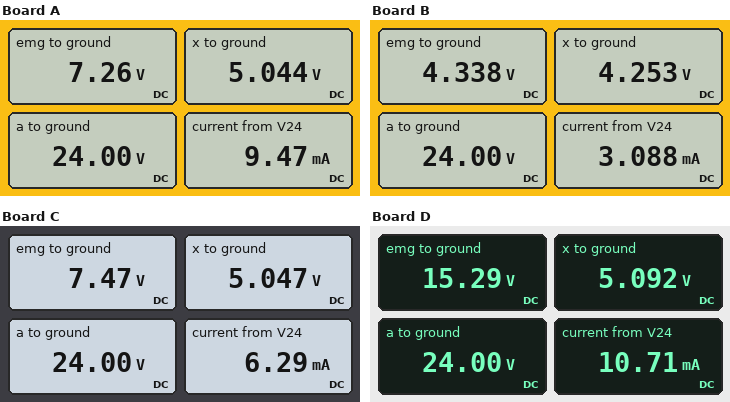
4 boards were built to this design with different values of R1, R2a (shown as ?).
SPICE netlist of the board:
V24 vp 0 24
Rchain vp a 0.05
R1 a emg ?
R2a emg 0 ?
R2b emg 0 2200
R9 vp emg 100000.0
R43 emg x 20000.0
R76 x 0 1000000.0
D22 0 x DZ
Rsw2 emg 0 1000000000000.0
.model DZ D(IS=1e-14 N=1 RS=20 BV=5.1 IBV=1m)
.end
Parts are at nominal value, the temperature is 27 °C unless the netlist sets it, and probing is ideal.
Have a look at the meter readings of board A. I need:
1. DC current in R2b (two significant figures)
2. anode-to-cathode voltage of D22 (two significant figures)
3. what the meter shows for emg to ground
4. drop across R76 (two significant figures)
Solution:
3.3 mA
-5.0 V
7.26 V
5.0 V
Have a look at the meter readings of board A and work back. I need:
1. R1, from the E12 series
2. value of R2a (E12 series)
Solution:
1.8 kΩ
1.2 kΩ
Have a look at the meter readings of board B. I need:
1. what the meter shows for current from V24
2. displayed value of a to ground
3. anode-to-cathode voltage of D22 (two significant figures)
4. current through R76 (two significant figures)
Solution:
3.088 mA
24.00 V
-4.3 V
4.3 µA
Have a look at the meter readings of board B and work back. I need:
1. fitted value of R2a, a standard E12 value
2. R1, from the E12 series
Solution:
3.9 kΩ
6.8 kΩ
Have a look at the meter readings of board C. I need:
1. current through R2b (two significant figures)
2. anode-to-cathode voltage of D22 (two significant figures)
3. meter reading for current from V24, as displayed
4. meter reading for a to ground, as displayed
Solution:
3.4 mA
-5.0 V
6.29 mA
24.00 V
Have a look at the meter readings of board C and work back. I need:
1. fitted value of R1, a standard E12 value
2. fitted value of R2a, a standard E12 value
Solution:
2.7 kΩ
2.7 kΩ
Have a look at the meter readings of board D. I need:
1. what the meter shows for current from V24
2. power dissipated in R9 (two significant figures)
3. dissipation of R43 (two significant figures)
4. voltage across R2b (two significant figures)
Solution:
10.71 mA
760 µW
5.2 mW
15 V
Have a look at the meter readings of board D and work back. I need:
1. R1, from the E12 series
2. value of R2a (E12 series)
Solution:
820 Ω
4.7 kΩ
